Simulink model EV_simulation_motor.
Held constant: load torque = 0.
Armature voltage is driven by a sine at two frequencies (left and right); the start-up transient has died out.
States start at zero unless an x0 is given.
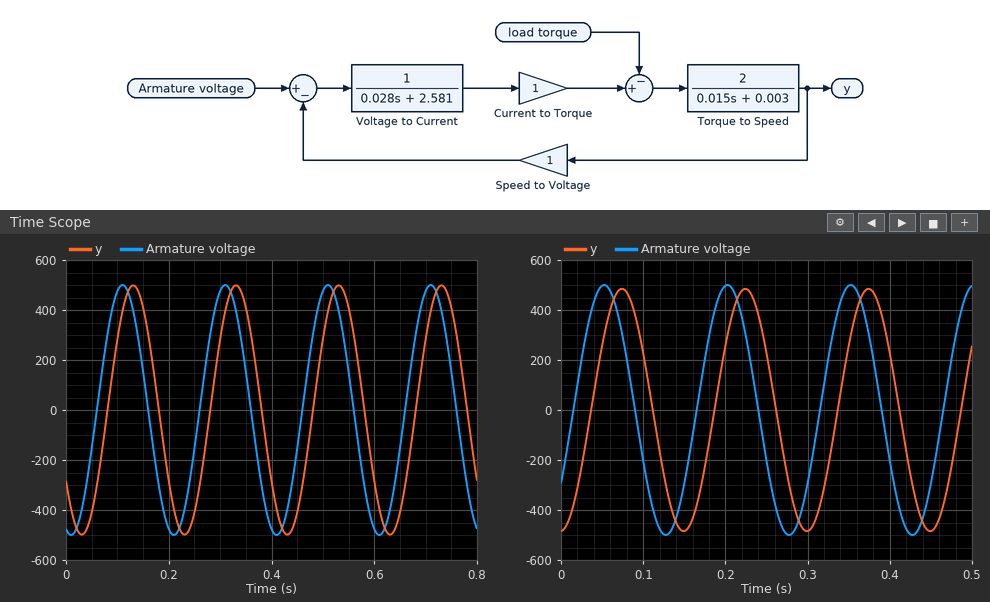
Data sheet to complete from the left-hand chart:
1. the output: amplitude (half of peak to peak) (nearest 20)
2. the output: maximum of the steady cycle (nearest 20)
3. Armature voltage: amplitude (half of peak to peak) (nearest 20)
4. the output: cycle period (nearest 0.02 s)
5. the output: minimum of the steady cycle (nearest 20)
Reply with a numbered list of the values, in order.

1. 500
2. 500
3. 500
4. 0.20 s
5. -500
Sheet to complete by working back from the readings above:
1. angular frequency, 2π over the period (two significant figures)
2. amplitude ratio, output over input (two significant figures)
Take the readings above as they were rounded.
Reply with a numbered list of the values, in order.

1. 31 rad/s
2. 1.0
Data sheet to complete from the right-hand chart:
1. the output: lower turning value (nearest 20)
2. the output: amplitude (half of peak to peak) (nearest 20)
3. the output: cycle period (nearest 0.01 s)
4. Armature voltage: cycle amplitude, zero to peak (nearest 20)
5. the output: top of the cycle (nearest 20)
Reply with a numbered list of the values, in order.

1. -480
2. 480
3. 0.15 s
4. 500
5. 480
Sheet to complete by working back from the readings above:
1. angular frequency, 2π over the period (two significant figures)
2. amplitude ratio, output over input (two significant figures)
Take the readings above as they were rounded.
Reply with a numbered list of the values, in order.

1. 42 rad/s
2. 0.96
